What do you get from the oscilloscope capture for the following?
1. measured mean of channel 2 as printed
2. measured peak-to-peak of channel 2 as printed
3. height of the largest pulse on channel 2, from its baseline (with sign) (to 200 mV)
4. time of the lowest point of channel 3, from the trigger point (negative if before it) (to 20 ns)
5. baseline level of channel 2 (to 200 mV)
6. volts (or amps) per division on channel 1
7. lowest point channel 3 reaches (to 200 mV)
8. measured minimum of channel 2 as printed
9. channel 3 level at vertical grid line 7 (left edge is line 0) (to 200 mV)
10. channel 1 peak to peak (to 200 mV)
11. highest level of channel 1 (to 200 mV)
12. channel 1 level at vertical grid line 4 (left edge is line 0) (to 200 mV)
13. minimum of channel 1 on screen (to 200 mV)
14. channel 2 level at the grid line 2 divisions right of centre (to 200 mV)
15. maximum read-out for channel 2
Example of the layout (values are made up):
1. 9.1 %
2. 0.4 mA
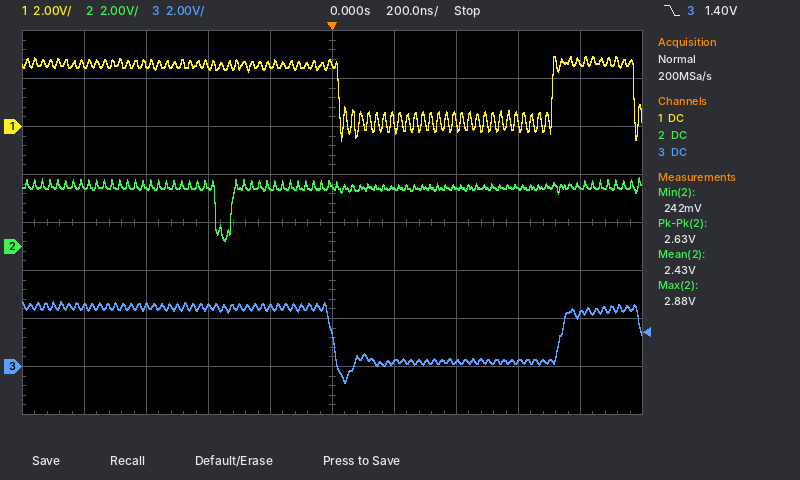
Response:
1. 2.43 V
2. 2.63 V
3. -2.2 V
4. +40 ns
5. 2.4 V
6. 2 V
7. -600 mV
8. 242 mV
9. 200 mV
10. 3.6 V
11. 3.0 V
12. 2.6 V
13. -600 mV
14. 2.4 V
15. 2.88 V
